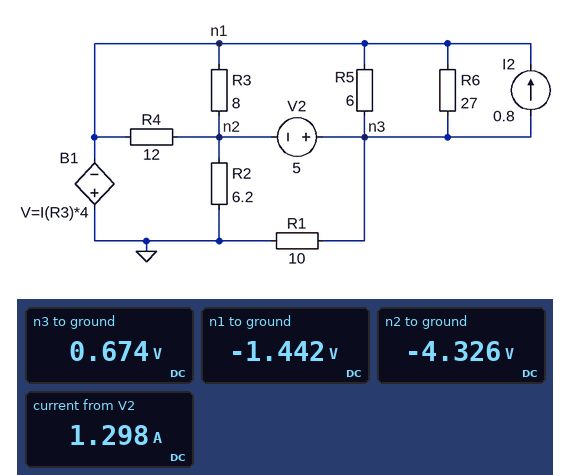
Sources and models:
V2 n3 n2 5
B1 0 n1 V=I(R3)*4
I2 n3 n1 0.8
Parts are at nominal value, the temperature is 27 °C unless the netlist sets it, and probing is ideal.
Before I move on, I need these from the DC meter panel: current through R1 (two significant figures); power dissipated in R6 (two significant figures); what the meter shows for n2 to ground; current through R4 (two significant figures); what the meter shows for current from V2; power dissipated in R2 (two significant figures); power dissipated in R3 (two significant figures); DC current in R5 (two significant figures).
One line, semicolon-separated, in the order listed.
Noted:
67 mA; 170 mW; -4.326 V; 240 mA; 1.298 A; 3.0 W; 1.0 W; 350 mA
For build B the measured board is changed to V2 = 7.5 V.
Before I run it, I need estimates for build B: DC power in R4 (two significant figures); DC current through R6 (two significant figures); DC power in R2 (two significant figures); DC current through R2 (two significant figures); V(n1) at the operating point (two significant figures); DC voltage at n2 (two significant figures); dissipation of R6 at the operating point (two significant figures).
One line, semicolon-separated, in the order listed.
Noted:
1.2 W; 140 mA; 5.3 W; 930 mA; -1.9 V; -5.7 V; 500 mW
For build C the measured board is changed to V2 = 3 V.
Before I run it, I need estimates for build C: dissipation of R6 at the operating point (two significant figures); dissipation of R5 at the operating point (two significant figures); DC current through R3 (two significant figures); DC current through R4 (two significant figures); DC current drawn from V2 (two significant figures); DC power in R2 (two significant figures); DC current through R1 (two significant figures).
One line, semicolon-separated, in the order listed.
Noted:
28 mW; 130 mW; 270 mA; 180 mA; 960 mA; 1.6 W; 19 mA
